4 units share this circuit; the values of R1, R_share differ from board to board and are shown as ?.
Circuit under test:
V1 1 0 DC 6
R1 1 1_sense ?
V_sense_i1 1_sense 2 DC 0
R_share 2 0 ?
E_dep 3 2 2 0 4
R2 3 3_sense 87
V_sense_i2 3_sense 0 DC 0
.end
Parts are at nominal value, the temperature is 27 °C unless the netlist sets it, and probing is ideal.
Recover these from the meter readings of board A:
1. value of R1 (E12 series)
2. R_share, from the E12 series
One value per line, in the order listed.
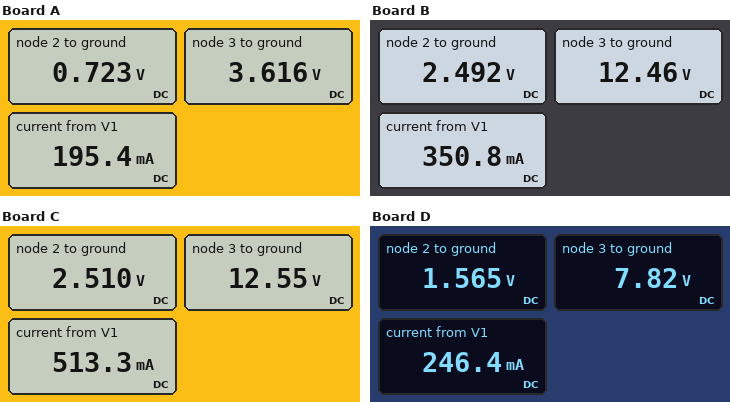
27 Ω
4.7 Ω
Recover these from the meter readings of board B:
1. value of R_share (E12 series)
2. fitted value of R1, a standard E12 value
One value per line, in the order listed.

12 Ω
10 Ω
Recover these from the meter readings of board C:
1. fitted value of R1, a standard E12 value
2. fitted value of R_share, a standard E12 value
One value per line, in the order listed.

6.8 Ω
6.8 Ω
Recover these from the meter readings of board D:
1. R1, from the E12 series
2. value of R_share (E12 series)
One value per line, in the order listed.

18 Ω
10 Ω
